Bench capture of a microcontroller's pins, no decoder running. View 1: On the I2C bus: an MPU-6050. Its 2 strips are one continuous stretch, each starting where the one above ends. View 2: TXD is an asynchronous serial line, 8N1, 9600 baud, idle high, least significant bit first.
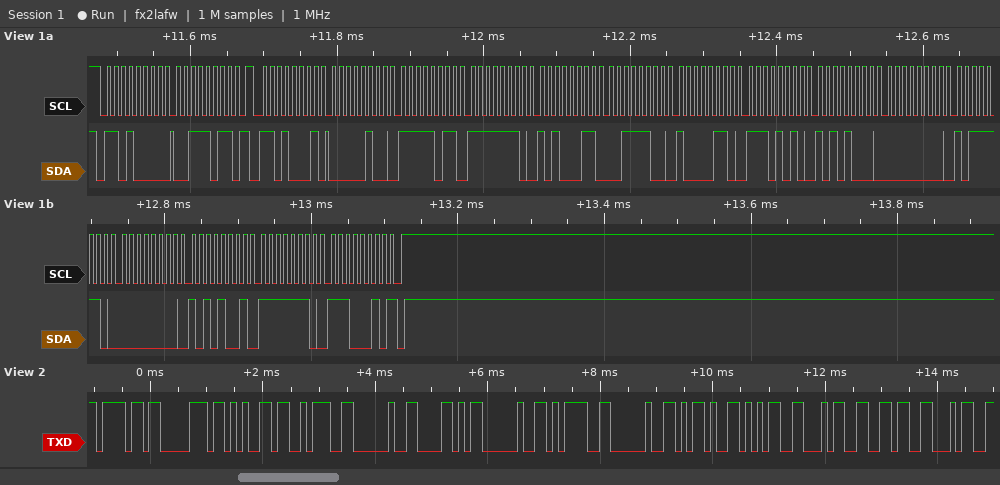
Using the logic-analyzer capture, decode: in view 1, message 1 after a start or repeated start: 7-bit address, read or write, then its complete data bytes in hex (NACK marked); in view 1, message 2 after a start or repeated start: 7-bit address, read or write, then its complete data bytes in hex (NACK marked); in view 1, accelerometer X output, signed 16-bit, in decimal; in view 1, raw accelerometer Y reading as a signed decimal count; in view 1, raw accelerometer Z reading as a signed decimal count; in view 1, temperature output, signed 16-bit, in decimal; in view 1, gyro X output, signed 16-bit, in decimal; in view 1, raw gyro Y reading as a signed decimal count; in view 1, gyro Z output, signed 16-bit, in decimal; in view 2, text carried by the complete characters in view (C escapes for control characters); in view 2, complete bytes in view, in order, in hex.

0x68 write: 3B
0x68 read: 04 FB FE A3 3C 86 EA A8 00 BE 00 A9 FE E2 NACK
1275
-349
15494
-5464
190
169
-286
"ope: X = -5464"
6F 70 65 3A 20 58 20 3D 20 2D 35 34 36 34
